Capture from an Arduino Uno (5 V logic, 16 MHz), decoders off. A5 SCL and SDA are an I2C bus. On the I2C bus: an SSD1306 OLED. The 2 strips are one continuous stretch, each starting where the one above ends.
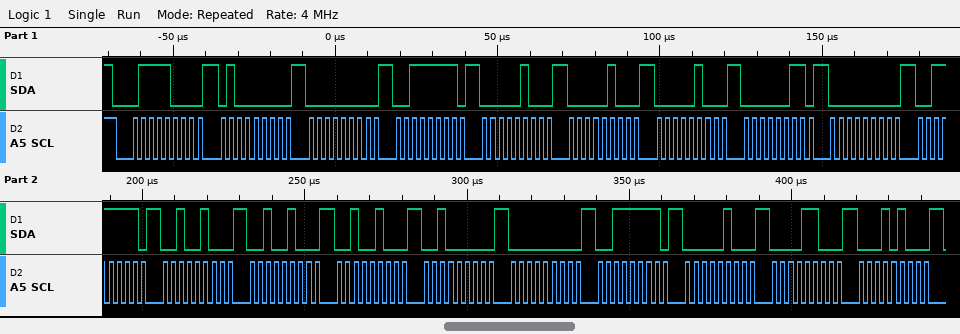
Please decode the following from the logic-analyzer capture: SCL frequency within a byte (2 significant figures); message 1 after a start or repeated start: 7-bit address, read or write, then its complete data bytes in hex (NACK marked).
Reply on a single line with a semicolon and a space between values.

400 kHz; 0x3C write: 40 00 3F 04 04 04 03 00 3F 24 24 24 20 00 3F 04 0C 14
